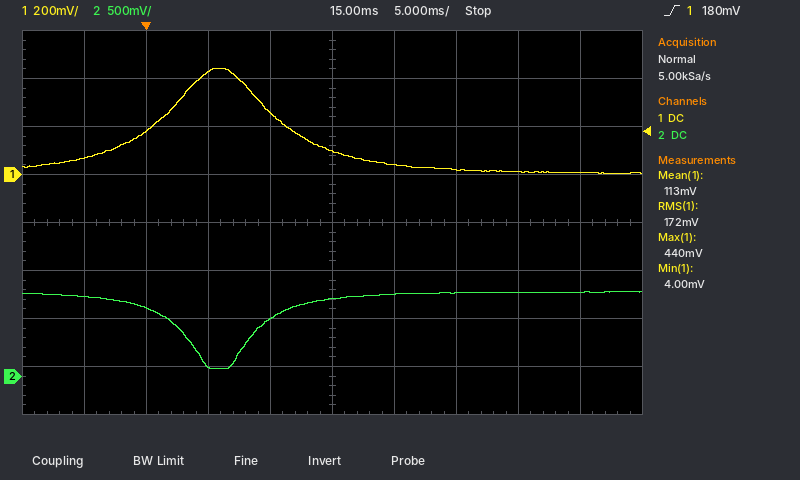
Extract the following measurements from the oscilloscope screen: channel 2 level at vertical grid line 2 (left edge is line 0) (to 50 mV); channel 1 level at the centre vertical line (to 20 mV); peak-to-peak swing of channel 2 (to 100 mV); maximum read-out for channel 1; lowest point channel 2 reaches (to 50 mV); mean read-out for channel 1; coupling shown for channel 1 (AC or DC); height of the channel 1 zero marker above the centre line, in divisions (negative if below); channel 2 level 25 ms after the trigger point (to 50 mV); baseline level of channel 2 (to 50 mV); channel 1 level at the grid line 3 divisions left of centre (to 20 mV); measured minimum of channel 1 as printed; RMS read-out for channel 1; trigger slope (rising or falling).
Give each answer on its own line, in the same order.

700 mV
100 mV
800 mV
440 mV
100 mV
113 mV
DC
+1.0 div
850 mV
850 mV
180 mV
4.00 mV
172 mV
rising
